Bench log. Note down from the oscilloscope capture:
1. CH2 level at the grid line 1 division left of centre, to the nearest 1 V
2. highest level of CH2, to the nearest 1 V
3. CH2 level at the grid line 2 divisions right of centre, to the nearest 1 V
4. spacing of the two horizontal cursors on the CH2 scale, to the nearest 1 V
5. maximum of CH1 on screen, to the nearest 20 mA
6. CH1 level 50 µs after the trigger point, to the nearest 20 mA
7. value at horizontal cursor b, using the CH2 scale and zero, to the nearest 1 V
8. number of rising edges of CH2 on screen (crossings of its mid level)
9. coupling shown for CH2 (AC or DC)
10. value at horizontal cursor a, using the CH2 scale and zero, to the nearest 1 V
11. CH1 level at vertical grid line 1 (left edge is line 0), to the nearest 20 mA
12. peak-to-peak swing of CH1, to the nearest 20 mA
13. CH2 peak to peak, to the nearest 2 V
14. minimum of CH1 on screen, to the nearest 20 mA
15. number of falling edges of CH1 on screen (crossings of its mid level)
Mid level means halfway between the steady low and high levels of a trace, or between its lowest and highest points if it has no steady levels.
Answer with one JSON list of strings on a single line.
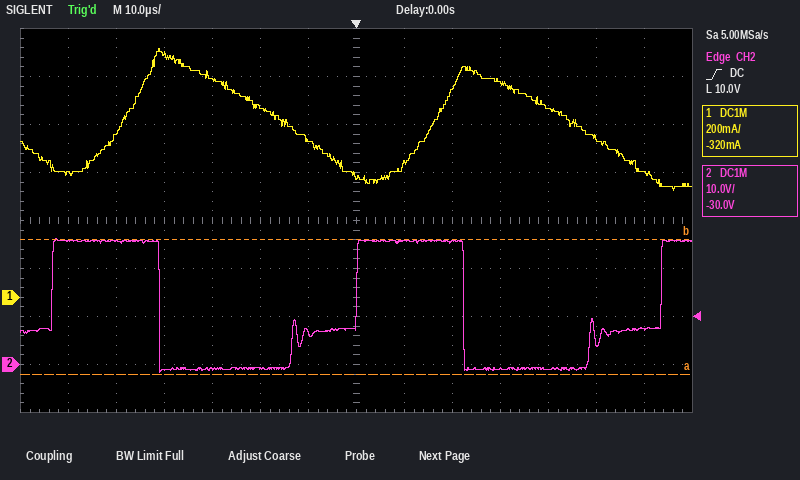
["7 V", "26 V", "26 V", "28 V", "1.04 A", "660 mA", "26 V", "3", "DC", "-2 V", "520 mA", "600 mA", "28 V", "440 mA", "2"]
